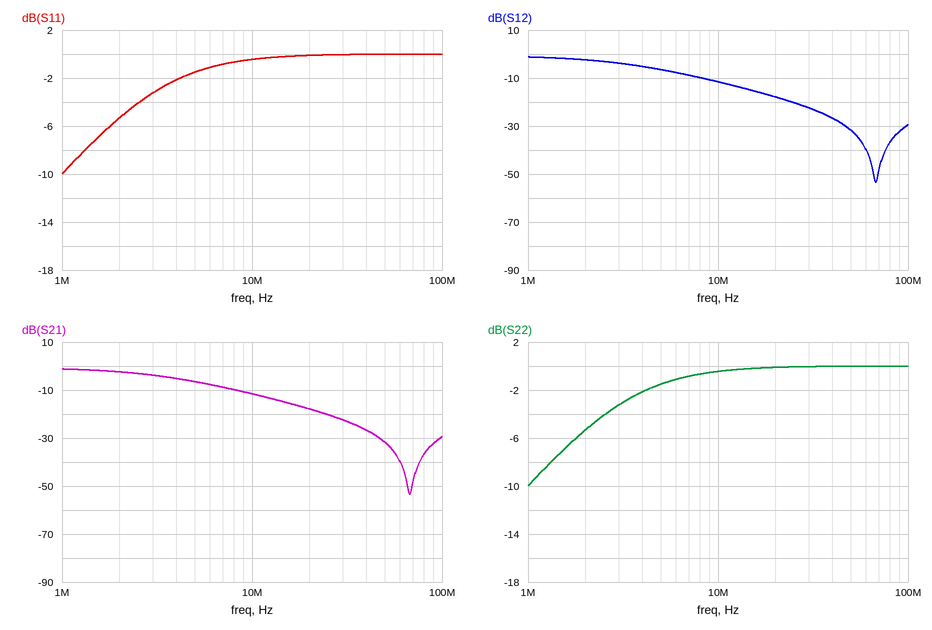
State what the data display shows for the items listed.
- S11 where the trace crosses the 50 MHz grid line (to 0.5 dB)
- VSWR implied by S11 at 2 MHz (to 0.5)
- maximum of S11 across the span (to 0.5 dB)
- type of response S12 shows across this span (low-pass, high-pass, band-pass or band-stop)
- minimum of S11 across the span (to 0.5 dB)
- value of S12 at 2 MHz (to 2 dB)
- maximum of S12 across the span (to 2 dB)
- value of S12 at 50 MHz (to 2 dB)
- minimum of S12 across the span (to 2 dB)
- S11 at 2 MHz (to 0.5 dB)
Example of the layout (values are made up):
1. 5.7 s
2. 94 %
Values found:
1. 0.0 dB
2. 3.5
3. 0.0 dB
4. low-pass
5. -10.0 dB
6. -2 dB
7. -2 dB
8. -32 dB
9. -54 dB
10. -5.5 dB
